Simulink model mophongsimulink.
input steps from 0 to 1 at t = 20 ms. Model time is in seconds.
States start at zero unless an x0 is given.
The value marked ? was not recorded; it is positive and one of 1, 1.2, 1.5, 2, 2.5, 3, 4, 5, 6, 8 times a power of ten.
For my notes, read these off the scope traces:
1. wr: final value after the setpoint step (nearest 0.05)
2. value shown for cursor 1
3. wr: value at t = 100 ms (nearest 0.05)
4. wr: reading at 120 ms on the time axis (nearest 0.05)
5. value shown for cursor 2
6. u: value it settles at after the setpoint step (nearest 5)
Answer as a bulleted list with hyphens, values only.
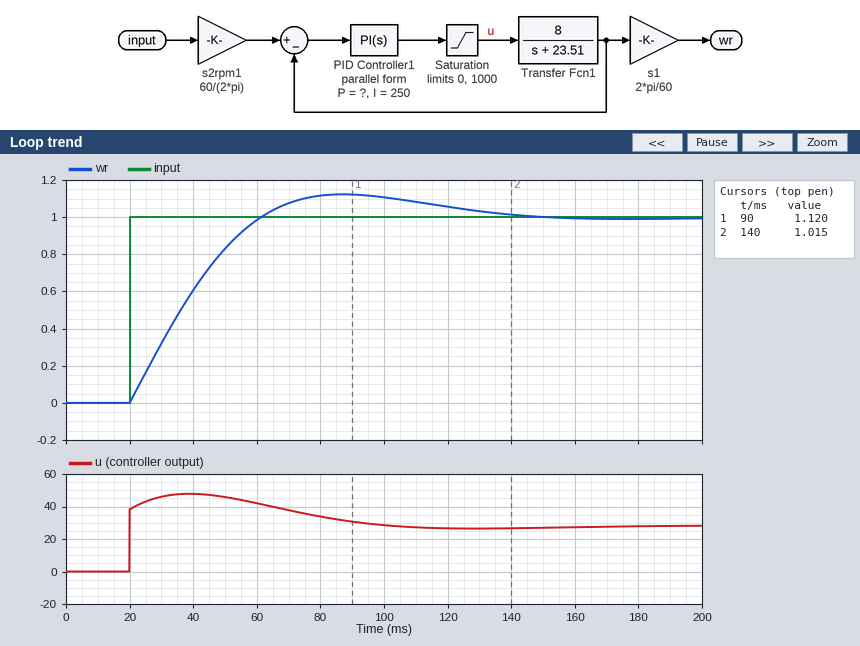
- 1.00
- 1.120
- 1.10
- 1.05
- 1.015
- 30
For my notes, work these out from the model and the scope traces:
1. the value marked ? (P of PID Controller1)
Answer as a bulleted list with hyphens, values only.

- 4
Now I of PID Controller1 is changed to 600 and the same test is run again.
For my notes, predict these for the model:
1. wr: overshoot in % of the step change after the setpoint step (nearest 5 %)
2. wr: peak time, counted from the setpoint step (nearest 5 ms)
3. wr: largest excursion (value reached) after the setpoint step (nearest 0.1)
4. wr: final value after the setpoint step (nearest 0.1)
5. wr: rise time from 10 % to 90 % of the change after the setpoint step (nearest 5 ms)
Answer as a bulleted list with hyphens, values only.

- 30 %
- 40 ms
- 1.3
- 1.0
- 20 ms
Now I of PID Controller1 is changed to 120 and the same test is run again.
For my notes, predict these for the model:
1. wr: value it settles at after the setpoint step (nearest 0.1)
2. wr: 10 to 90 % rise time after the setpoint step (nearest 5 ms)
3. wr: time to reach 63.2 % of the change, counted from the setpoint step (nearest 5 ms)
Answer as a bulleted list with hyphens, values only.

- 1.0
- 55 ms
- 30 ms
